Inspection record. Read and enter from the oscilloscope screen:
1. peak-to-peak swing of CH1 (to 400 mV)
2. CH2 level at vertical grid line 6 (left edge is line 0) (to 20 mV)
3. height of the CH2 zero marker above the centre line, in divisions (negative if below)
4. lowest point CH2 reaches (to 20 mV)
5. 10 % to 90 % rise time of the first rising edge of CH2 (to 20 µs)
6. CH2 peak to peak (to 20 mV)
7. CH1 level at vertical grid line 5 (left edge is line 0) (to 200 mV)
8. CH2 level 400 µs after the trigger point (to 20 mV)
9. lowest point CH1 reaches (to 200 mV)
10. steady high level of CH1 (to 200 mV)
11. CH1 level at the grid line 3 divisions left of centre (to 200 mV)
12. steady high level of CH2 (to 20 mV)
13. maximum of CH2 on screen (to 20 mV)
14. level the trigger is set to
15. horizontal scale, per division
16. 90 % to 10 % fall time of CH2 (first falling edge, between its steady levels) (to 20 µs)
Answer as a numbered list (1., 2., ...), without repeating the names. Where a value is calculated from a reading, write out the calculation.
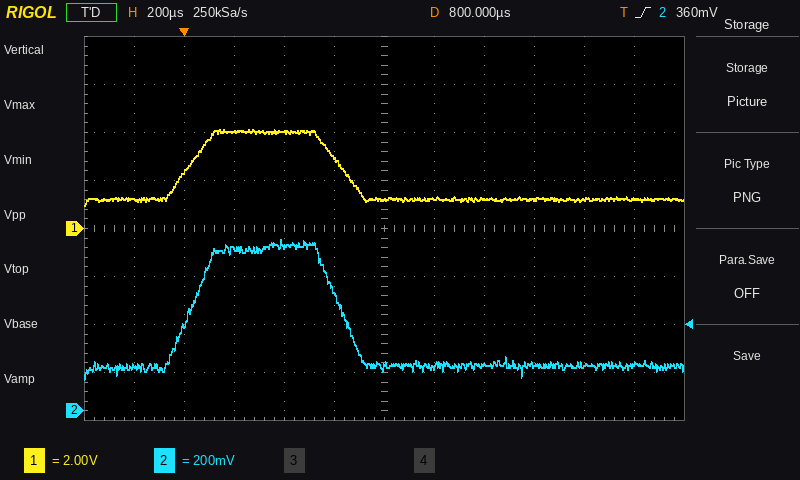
1. 3.2 V
2. 180 mV
3. -3.8 div
4. 140 mV
5. 160 µs
6. 720 mV − (140 mV) = 580 mV
7. 3.0 V
8. 700 mV
9. 1.0 V
10. 4.0 V
11. 4.0 V
12. 680 mV
13. 720 mV
14. 360 mV
15. 200 µs
16. 160 µs
